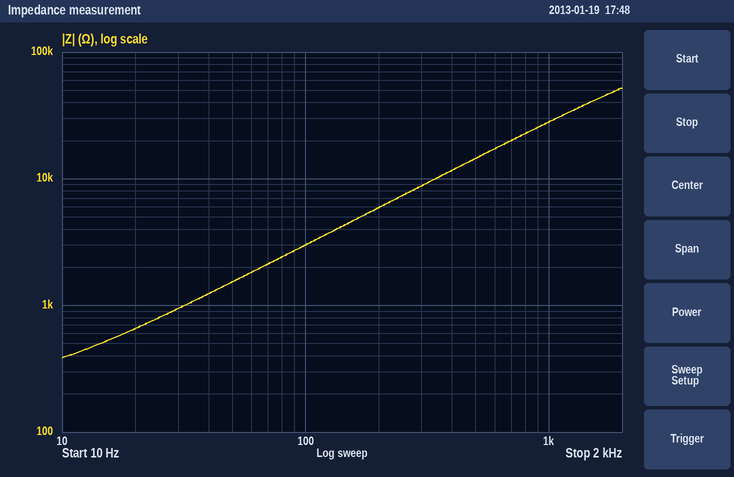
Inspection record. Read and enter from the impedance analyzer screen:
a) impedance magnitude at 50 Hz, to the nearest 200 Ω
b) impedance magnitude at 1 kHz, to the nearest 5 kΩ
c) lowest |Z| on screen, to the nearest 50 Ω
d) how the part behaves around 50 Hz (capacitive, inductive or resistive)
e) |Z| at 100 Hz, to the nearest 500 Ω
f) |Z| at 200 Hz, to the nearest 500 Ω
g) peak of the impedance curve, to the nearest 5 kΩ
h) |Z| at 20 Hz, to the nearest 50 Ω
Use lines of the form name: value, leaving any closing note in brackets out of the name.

impedance magnitude at 50 Hz, to the nearest 200 Ω: 1.6 kΩ
impedance magnitude at 1 kHz, to the nearest 5 kΩ: 30 kΩ
lowest |Z| on screen, to the nearest 50 Ω: 400 Ω
how the part behaves around 50 Hz: inductive
|Z| at 100 Hz, to the nearest 500 Ω: 3.0 kΩ
|Z| at 200 Hz, to the nearest 500 Ω: 6.0 kΩ
peak of the impedance curve, to the nearest 5 kΩ: 50 kΩ
|Z| at 20 Hz, to the nearest 50 Ω: 650 Ω
